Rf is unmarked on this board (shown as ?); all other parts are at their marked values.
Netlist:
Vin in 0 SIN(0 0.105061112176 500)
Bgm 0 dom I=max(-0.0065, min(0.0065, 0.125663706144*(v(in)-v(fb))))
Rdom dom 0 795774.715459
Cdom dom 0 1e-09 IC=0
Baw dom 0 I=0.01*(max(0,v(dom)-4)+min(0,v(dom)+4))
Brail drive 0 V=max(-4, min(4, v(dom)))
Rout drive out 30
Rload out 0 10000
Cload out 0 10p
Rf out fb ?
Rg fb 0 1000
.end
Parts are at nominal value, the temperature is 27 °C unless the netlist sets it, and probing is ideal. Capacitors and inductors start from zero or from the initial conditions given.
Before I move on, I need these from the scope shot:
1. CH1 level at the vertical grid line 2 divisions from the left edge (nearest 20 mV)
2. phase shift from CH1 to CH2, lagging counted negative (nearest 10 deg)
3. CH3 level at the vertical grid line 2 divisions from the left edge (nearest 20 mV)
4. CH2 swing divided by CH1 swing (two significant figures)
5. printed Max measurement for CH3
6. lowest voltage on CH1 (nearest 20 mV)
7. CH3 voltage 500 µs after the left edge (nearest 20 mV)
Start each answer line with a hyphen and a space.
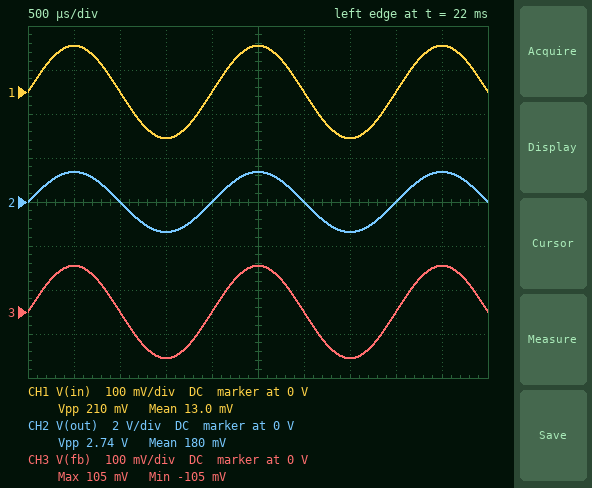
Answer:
- 0 V
- 0 deg
- 0 V
- 13
- 105 mV
- -100 mV
- 100 mV
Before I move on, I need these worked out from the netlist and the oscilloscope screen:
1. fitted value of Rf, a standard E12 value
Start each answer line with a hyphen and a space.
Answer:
- 12 kΩ
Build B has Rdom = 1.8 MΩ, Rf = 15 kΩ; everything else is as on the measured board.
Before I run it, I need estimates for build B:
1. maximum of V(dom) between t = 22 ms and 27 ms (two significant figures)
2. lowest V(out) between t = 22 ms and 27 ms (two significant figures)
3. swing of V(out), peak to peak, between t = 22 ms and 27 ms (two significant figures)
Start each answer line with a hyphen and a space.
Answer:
- 1.7 V
- -1.7 V
- 3.4 V
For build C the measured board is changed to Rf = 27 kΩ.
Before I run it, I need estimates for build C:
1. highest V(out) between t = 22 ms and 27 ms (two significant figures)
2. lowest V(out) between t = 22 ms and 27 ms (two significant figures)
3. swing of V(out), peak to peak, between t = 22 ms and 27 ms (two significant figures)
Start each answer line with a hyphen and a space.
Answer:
- 2.9 V
- -2.9 V
- 5.9 V
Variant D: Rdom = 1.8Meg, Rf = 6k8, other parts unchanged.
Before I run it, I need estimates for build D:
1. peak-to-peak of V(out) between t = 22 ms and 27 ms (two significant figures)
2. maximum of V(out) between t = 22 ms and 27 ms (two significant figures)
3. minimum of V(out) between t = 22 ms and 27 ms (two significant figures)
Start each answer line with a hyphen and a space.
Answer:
- 1.6 V
- 820 mV
- -820 mV
